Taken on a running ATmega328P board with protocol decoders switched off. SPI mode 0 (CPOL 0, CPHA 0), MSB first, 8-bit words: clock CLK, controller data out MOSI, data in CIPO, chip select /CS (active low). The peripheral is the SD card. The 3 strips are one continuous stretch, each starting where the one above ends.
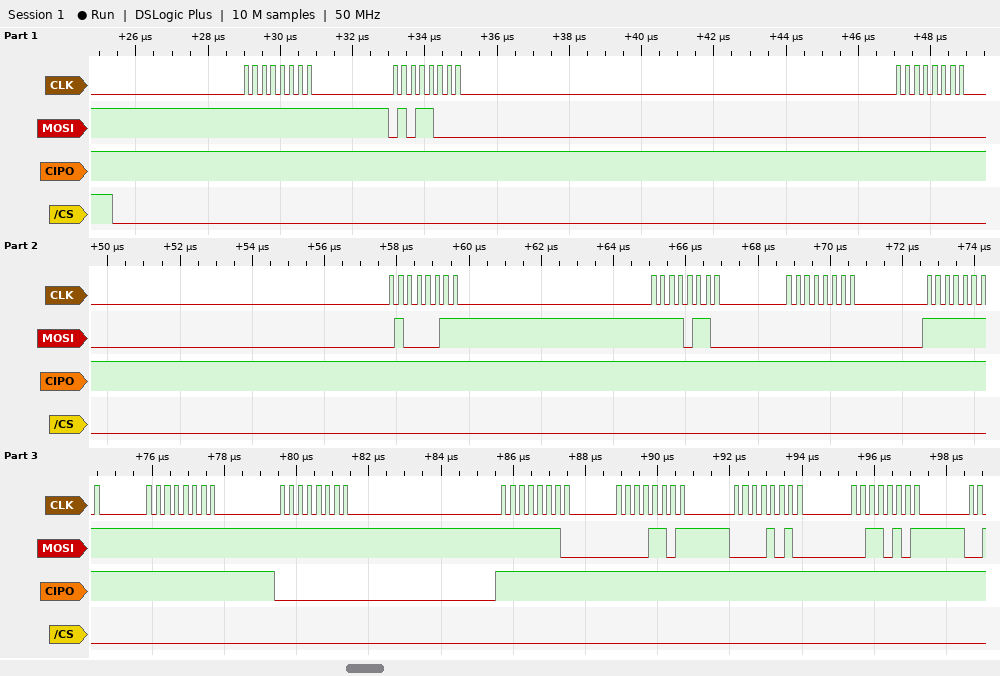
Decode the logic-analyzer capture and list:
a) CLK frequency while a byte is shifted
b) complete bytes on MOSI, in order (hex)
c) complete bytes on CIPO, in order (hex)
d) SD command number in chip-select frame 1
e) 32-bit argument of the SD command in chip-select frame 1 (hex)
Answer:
4 MHz
FF 58 00 43 F6 00 FF FF FF FE 0D 0A 35
FF FF FF FF FF FF FF FF 00 FF FF FF FF
CMD24
0x0043F600
